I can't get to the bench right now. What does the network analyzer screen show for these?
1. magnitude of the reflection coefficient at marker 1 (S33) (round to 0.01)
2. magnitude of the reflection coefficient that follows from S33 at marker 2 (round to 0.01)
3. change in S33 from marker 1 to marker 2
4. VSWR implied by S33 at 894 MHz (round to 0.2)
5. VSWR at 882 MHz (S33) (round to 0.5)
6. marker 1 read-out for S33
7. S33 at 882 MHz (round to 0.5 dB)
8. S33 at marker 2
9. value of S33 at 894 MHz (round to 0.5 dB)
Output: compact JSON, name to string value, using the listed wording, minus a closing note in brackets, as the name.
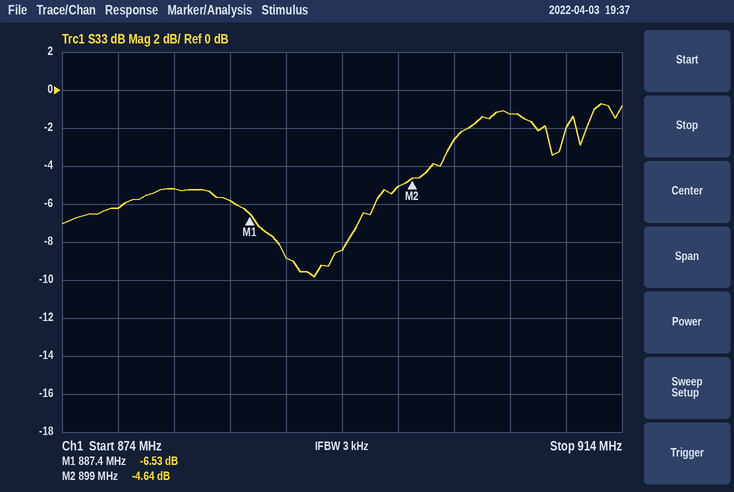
{"magnitude of the reflection coefficient at marker 1 (S33)": "0.47", "magnitude of the reflection coefficient that follows from S33 at marker 2": "0.59", "change in S33 from marker 1 to marker 2": "1.89 dB", "VSWR implied by S33 at 894 MHz": "2.2", "VSWR at 882 MHz (S33)": "3.5", "marker 1 read-out for S33": "-6.53 dB", "S33 at 882 MHz": "-5.0 dB", "S33 at marker 2": "-4.64 dB", "value of S33 at 894 MHz": "-8.5 dB"}
